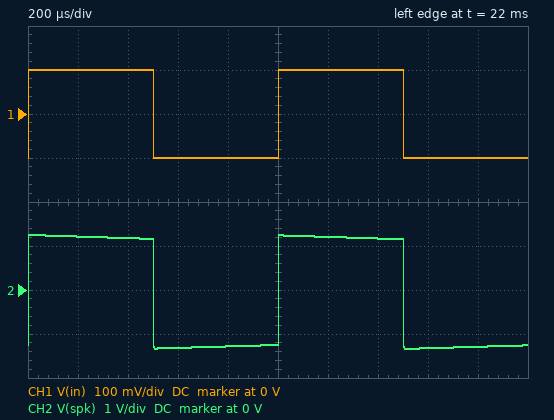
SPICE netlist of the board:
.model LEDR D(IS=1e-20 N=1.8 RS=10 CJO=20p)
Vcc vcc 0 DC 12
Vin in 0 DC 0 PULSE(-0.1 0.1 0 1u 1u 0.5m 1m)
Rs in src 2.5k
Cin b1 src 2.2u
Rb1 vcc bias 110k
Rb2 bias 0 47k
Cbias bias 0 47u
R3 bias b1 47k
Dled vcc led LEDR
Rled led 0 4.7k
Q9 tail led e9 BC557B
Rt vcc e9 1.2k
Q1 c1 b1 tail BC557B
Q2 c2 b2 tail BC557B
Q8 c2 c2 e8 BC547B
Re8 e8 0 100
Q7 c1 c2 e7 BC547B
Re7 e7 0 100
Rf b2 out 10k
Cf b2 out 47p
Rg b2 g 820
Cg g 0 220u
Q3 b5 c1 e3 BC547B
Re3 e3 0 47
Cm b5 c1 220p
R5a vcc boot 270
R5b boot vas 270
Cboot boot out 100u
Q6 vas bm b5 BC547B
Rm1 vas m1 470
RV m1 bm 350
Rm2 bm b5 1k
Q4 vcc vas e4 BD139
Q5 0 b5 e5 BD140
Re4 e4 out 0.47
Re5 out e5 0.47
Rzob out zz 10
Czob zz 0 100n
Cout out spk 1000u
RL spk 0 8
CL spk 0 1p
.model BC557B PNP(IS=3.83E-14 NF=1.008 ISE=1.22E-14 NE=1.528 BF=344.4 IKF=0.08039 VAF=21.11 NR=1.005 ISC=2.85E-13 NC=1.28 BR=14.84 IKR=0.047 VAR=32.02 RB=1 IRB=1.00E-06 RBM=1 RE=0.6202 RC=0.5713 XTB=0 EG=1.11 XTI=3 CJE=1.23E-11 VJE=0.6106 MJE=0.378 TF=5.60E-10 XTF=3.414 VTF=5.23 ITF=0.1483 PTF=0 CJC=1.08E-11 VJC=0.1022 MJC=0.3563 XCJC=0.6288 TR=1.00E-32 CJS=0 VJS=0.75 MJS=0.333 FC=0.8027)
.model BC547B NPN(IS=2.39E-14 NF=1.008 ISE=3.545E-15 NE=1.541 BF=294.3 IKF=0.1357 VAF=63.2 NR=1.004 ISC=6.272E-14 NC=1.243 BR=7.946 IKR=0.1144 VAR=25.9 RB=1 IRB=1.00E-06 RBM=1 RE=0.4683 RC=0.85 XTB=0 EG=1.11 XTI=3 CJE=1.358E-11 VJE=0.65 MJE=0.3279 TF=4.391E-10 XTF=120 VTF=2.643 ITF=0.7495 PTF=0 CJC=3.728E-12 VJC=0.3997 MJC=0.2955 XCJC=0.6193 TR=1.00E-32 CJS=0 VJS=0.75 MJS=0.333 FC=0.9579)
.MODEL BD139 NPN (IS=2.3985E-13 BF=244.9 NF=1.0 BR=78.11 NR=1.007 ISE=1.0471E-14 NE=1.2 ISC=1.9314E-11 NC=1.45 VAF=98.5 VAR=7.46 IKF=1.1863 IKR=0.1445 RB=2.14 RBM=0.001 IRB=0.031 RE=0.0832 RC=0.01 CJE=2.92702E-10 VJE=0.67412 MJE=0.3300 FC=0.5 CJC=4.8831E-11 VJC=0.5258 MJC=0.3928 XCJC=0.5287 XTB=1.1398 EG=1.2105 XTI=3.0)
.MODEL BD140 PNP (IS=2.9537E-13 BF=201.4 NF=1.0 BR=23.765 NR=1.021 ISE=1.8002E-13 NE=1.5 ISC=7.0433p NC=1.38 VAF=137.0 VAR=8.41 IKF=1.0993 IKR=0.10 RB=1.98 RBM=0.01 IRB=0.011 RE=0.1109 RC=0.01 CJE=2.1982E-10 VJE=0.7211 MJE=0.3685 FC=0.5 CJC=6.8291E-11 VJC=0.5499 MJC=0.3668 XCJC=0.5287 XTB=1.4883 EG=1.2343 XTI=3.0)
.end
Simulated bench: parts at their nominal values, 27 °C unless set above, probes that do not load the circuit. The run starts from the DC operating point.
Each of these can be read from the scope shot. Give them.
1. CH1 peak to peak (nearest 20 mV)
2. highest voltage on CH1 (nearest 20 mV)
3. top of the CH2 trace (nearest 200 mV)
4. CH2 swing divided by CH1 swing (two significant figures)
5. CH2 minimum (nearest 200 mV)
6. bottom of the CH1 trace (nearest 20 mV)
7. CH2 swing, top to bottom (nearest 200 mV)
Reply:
200 mV
100 mV
1.2 V
13
-1.4 V
-100 mV
2.6 V
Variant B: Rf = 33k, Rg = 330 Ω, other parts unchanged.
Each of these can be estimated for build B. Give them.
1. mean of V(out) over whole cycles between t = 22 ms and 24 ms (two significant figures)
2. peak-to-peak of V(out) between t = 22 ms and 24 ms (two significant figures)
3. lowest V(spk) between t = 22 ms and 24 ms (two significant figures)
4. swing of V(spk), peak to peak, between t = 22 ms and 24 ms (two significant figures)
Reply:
6.8 V
9.6 V
-4.8 V
9.9 V
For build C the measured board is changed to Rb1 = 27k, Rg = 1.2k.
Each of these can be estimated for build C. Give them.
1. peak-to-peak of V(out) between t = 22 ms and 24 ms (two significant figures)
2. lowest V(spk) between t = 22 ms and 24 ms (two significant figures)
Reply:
1.8 V
-940 mV
